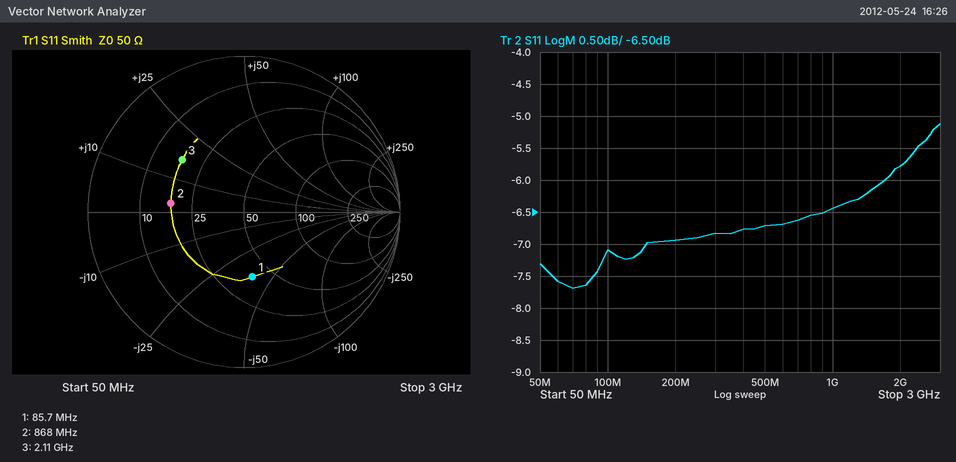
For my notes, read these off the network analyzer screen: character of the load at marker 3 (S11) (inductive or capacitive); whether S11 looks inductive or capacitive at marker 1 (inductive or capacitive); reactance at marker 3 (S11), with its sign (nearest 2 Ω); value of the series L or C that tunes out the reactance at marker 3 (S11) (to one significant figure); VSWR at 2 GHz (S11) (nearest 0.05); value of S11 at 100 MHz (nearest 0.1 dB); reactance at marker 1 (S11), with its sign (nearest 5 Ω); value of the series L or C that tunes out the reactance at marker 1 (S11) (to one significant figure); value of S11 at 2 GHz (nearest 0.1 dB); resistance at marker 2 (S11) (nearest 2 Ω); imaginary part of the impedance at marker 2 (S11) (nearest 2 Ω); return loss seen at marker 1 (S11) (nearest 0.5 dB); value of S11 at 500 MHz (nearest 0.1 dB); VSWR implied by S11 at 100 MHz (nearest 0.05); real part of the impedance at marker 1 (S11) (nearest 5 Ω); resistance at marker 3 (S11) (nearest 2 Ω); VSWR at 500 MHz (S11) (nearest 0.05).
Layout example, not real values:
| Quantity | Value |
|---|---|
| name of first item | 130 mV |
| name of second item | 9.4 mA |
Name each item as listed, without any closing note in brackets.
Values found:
| Quantity | Value |
|---|---|
| character of the load at marker 3 (S11) | inductive |
| whether S11 looks inductive or capacitive at marker 1 | capacitive |
| reactance at marker 3 (S11), with its sign | +16 Ω |
| value of the series L or C that tunes out the reactance at marker 3 (S11) | 5 pF |
| VSWR at 2 GHz (S11) | 3.10 |
| value of S11 at 100 MHz | -7.1 dB |
| reactance at marker 1 (S11), with its sign | -40 Ω |
| value of the series L or C that tunes out the reactance at marker 1 (S11) | 70 nH |
| value of S11 at 2 GHz | -5.8 dB |
| resistance at marker 2 (S11) | 18 Ω |
| imaginary part of the impedance at marker 2 (S11) | +2 Ω |
| return loss seen at marker 1 (S11) | 7.5 dB |
| value of S11 at 500 MHz | -6.7 dB |
| VSWR implied by S11 at 100 MHz | 2.60 |
| real part of the impedance at marker 1 (S11) | 40 Ω |
| resistance at marker 3 (S11) | 18 Ω |
| VSWR at 500 MHz (S11) | 2.70 |
